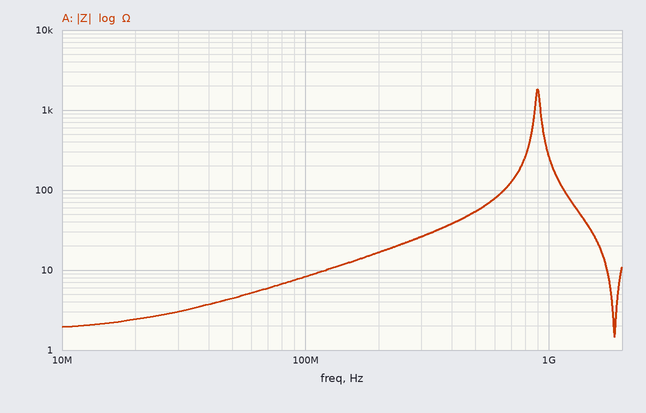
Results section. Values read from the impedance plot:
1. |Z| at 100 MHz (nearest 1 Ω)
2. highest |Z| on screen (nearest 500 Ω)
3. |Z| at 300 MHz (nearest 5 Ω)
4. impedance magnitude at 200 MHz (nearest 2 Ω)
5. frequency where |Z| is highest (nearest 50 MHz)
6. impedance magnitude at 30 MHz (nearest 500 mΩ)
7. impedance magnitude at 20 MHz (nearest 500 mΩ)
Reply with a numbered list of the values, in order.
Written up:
1. 8 Ω
2. 2.0 kΩ
3. 25 Ω
4. 16 Ω
5. 900 MHz
6. 3.0 Ω
7. 2.5 Ω
